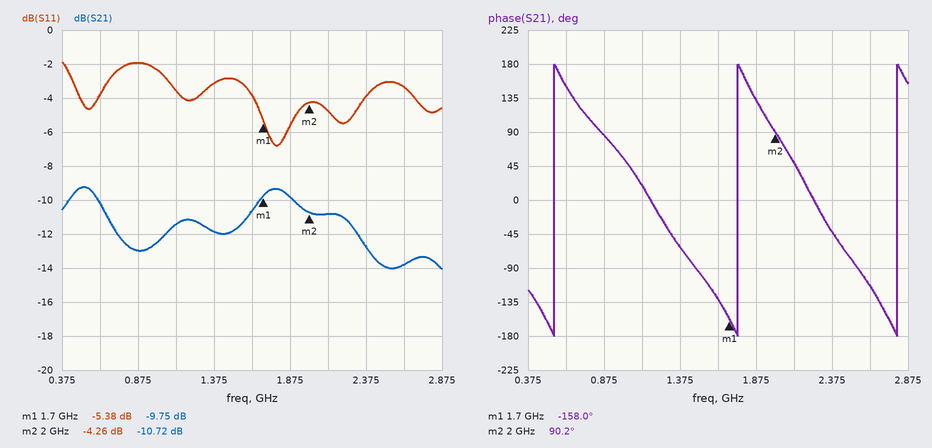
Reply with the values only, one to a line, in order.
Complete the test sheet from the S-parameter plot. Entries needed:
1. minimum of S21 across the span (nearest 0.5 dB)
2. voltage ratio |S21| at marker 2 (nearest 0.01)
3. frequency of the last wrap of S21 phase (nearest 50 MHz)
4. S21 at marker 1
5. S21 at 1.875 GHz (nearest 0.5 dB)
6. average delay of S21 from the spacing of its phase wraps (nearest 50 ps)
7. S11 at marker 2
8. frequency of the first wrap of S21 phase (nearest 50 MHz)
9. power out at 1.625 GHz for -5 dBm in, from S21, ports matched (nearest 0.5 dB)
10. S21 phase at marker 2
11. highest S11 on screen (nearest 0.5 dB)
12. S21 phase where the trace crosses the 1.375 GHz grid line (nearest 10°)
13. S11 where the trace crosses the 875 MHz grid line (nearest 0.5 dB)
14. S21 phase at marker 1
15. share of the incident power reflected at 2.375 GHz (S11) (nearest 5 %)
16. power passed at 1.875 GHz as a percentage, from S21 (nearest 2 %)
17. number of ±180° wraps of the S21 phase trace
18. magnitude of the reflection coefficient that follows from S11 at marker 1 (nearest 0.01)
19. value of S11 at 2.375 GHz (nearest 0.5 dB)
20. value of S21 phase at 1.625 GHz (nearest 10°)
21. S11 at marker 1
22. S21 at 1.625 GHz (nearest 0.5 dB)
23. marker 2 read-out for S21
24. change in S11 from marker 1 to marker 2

-14.0 dB
0.29
2.80 GHz
-9.75 dB
-10.0 dB
900 ps
-4.26 dB
550 MHz
-15.5 dBm
90.2°
-2.0 dB
-60°
-2.0 dB
-158.0°
40 %
10 %
3
0.54
-4.0 dB
-130°
-5.38 dB
-10.5 dB
-10.72 dB
1.12 dB
